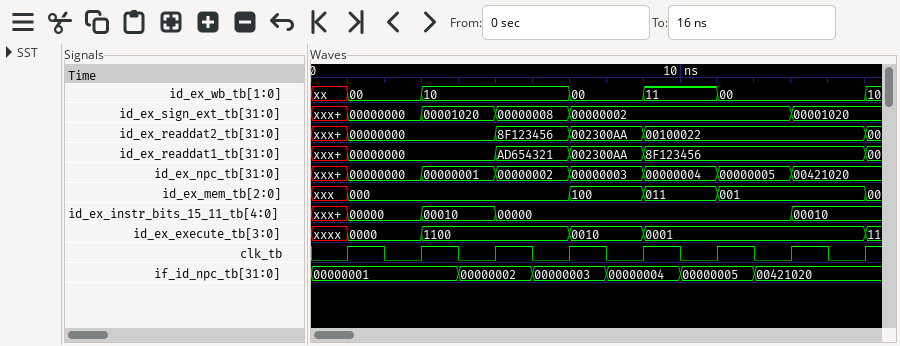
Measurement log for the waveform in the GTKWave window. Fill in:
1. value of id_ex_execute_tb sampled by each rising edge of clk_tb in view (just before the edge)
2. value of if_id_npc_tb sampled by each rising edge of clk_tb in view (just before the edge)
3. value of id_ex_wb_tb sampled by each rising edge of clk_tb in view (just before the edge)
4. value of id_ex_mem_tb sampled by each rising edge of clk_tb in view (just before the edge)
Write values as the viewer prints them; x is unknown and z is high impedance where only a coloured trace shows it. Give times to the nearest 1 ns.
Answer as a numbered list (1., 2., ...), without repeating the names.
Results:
1. xxxx, 0000, 1100, 1100, 0010, 0001, 0001, 0001
2. 00000001, 00000001, 00000002, 00000003, 00000004, 00000005, 00421020, 00421020
3. xx, 00, 10, 10, 00, 11, 00, 00
4. xxx, 000, 000, 000, 100, 011, 001, 001
